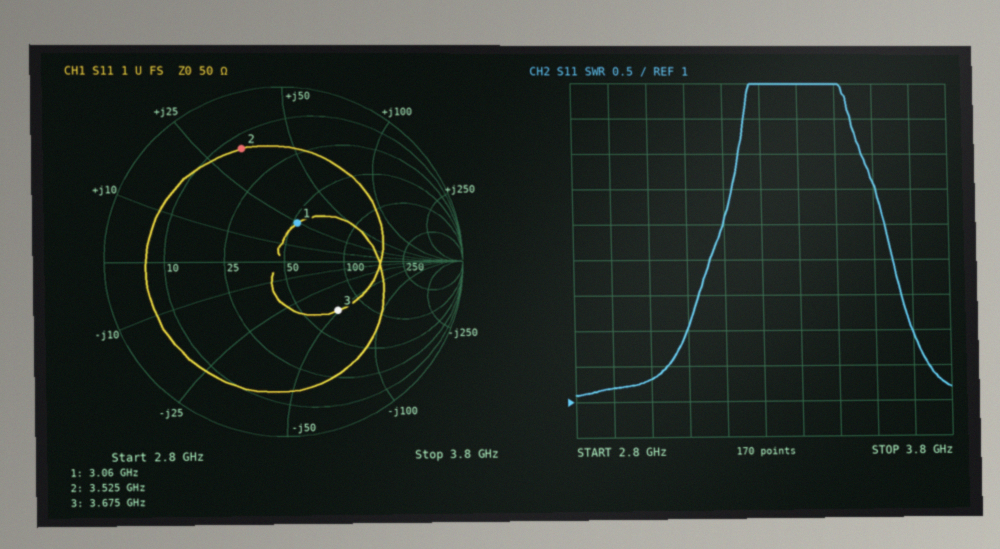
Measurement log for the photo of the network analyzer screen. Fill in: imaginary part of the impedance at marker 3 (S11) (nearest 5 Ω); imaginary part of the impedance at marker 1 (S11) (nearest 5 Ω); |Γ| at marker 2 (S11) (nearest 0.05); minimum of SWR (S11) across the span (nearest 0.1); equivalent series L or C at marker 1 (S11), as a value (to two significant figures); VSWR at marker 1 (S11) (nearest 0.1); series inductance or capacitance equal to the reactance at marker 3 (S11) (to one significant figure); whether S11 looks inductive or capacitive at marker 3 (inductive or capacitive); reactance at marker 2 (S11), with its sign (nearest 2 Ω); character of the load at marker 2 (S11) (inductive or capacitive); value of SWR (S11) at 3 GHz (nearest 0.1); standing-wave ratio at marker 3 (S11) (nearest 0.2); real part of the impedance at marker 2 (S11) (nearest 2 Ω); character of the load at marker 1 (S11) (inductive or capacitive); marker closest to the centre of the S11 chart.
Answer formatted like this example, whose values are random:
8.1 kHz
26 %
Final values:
-50 Ω
+25 Ω
0.70
1.1
1.3 nH
1.6
900 fF
capacitive
+34 Ω
inductive
1.3
2.4
14 Ω
inductive
marker 1
